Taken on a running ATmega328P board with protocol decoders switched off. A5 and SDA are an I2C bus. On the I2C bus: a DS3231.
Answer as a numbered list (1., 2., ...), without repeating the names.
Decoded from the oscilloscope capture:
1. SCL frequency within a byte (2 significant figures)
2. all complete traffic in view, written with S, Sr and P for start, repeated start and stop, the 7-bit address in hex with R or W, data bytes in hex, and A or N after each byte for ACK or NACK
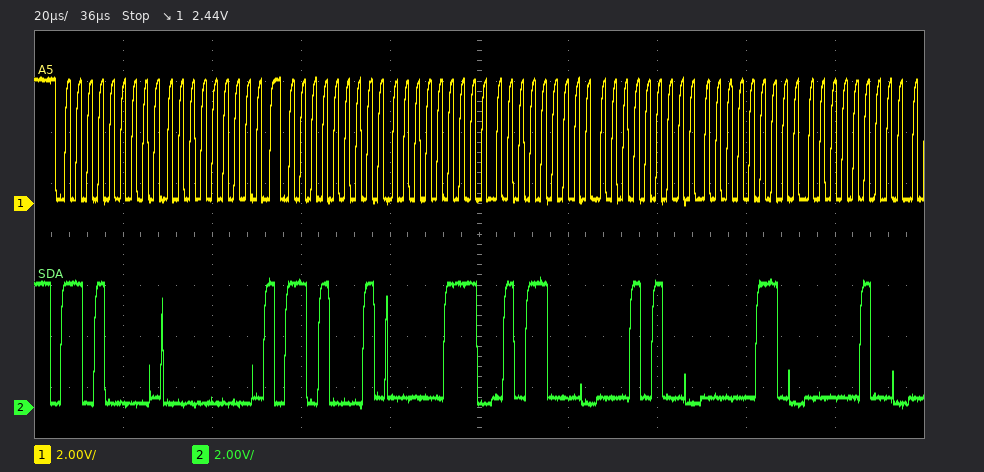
1. 400 kHz
2. S 68W A 00 A Sr 68R A 07 A 58 A 14 A 06 A 04 A
